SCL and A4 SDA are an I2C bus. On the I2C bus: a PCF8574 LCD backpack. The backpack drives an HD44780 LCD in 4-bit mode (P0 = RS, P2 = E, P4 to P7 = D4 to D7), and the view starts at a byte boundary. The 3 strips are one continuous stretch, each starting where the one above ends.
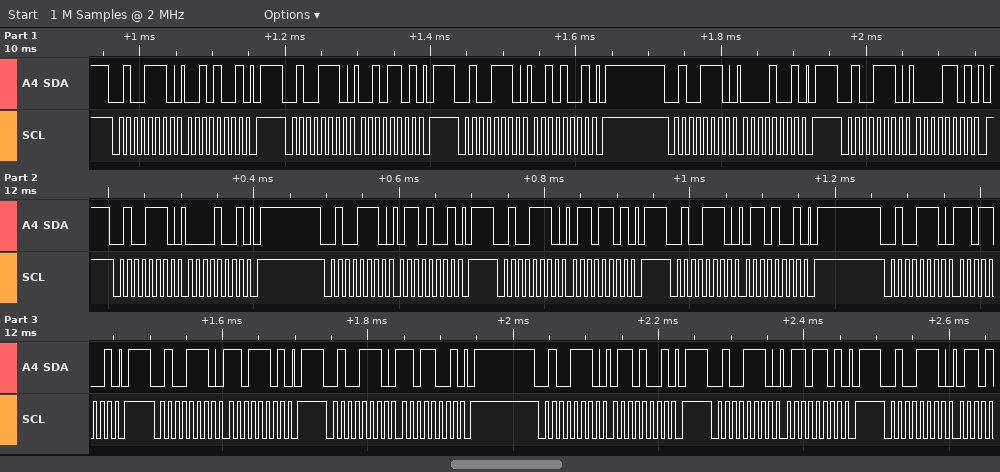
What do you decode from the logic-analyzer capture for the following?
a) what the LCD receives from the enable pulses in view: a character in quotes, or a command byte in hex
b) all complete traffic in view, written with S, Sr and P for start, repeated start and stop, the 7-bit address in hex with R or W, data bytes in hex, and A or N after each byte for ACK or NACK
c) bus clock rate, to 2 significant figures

' ' 'm'
S 27W A 29 A P S 27W A 2D A P S 27W A 29 A P S 27W A 09 A P S 27W A 0D A P S 27W A 09 A P S 27W A 69 A P S 27W A 6D A P S 27W A 69 A P S 27W A D9 A P S 27W A DD A P S 27W A D9 A P S 27W A 69 A P S 27W A 6D A P S 27W A
100 kHz
